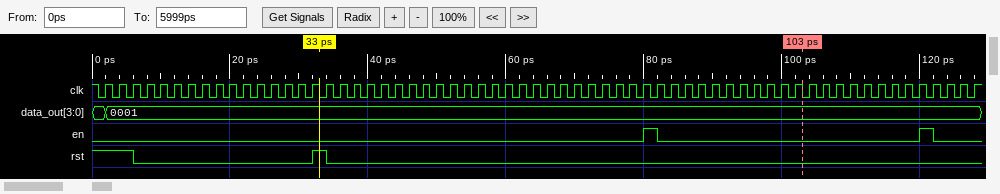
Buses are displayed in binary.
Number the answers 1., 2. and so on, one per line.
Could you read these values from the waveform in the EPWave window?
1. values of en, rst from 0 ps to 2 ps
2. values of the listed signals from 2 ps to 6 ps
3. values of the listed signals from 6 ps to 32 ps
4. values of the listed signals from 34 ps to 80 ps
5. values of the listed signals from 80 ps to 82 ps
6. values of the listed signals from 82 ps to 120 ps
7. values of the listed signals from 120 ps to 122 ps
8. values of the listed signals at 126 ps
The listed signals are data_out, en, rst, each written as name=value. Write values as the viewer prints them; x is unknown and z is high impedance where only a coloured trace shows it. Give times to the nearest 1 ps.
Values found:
1. en=0, rst=1
2. data_out=0001, en=0, rst=1
3. data_out=0001, en=0, rst=0
4. data_out=0001, en=0, rst=0
5. data_out=0001, en=1, rst=0
6. data_out=0001, en=0, rst=0
7. data_out=0001, en=1, rst=0
8. data_out=0001, en=0, rst=0
